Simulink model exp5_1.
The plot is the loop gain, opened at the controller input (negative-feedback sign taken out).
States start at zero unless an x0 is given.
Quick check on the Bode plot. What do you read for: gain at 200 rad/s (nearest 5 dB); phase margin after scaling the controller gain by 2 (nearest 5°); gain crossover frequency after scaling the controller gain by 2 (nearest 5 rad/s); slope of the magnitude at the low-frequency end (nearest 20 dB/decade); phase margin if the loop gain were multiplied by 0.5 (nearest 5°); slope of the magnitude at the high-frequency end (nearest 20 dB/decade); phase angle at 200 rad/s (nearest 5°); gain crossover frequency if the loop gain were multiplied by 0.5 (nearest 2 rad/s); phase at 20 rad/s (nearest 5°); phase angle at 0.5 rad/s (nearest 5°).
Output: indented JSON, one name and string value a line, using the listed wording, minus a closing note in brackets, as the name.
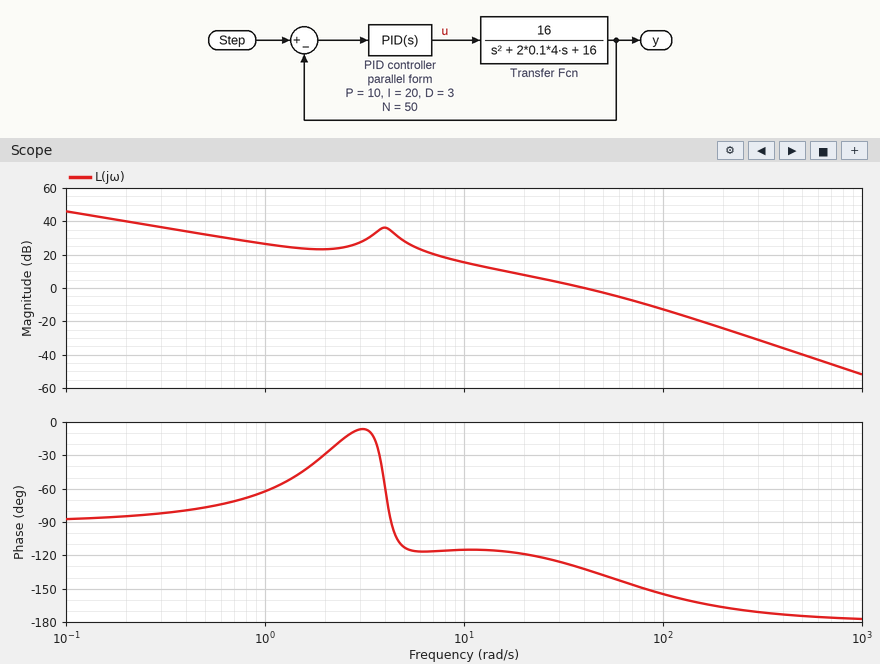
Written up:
{
  "gain at 200 rad/s": "-25 dB",
  "phase margin after scaling the controller gain by 2": "35°",
  "gain crossover frequency after scaling the controller gain by 2": "65 rad/s",
  "slope of the magnitude at the low-frequency end": "-20 dB/decade",
  "phase margin if the loop gain were multiplied by 0.5": "60°",
  "slope of the magnitude at the high-frequency end": "-40 dB/decade",
  "phase angle at 200 rad/s": "-165°",
  "gain crossover frequency if the loop gain were multiplied by 0.5": "24 rad/s",
  "phase at 20 rad/s": "-120°",
  "phase angle at 0.5 rad/s": "-75°"
}
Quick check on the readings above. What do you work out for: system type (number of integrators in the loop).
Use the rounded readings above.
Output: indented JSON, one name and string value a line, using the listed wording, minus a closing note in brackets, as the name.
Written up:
{
  "system type": "1"
}
